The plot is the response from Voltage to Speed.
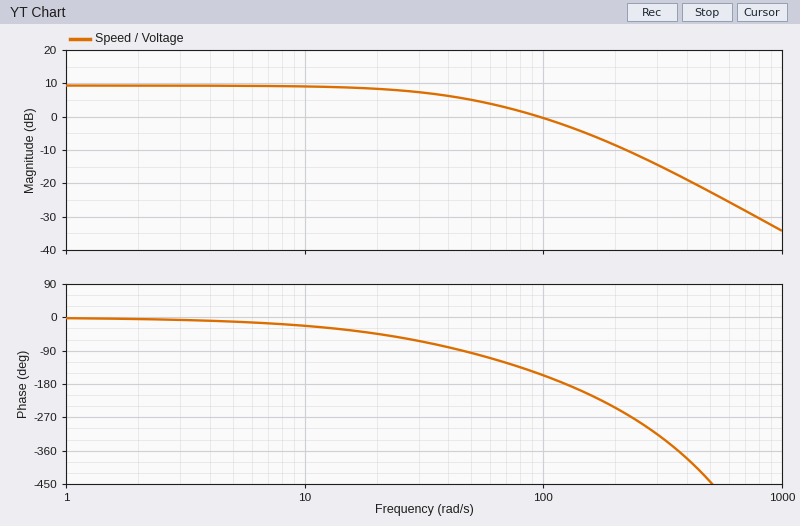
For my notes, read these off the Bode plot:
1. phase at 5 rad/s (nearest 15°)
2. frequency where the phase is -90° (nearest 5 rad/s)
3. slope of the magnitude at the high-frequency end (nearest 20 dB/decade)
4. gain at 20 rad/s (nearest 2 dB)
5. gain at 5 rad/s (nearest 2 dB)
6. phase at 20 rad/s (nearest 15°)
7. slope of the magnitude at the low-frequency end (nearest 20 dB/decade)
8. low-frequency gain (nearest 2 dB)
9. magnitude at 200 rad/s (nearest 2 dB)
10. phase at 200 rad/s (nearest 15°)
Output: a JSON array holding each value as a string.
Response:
["-15°", "45 rad/s", "-40 dB/decade", "8 dB", "10 dB", "-45°", "0 dB/decade", "10 dB", "-8 dB", "-240°"]
